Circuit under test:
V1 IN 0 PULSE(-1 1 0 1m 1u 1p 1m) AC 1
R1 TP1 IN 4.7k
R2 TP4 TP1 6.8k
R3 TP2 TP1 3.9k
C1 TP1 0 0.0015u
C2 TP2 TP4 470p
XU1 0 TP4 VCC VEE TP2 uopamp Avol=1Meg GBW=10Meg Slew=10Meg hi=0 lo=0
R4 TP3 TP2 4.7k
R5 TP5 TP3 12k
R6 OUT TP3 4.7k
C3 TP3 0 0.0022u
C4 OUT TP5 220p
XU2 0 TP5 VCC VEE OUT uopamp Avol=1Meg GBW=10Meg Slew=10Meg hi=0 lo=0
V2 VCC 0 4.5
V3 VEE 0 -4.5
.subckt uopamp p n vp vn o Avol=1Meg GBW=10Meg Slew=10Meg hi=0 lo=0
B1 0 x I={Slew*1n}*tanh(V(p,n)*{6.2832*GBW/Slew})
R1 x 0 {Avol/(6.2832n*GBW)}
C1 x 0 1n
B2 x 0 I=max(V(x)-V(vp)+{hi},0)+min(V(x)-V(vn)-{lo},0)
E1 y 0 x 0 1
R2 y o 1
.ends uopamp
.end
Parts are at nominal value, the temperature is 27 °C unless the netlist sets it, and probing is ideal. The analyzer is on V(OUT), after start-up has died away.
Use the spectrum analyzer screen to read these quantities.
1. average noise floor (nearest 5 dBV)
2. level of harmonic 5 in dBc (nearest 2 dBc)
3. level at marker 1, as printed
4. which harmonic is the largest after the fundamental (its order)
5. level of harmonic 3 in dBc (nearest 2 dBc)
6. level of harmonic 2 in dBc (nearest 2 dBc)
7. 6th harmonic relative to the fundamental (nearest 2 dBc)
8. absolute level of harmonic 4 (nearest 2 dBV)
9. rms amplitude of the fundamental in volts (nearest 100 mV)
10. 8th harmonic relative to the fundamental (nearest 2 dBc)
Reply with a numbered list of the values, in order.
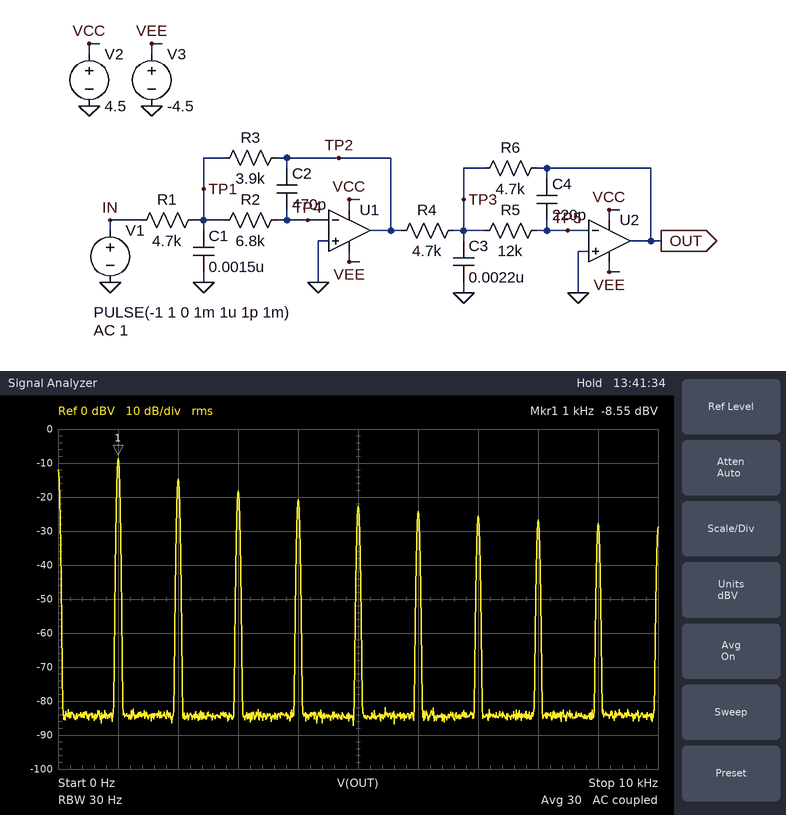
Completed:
1. -85 dBV
2. -14 dBc
3. -8.55 dBV
4. 2
5. -10 dBc
6. -6 dBc
7. -16 dBc
8. -20 dBV
9. 400 mV
10. -18 dBc
